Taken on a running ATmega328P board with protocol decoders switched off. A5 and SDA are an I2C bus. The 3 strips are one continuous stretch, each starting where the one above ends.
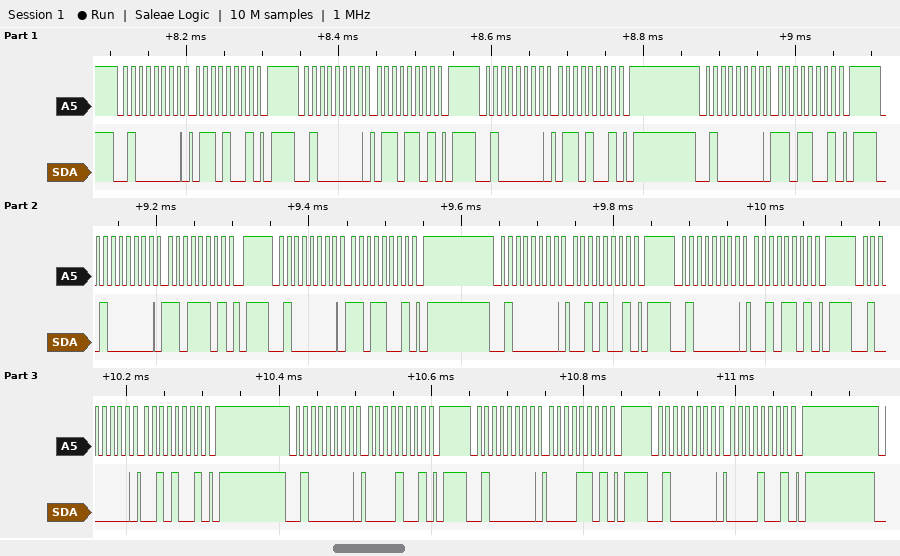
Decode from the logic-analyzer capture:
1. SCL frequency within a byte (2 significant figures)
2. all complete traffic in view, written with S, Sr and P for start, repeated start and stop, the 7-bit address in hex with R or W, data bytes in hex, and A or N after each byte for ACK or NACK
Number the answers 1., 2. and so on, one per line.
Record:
1. 100 kHz
2. S 20W A 69 A P S 20W A 6D A P S 20W A 69 A P S 20W A D9 A P S 20W A DD A P S 20W A D9 A P S 20W A 29 A P S 20W A 2D A P S 20W A 29 A P S 20W A 09 A P S 20W A 0D A P S 20W A 09 A P
